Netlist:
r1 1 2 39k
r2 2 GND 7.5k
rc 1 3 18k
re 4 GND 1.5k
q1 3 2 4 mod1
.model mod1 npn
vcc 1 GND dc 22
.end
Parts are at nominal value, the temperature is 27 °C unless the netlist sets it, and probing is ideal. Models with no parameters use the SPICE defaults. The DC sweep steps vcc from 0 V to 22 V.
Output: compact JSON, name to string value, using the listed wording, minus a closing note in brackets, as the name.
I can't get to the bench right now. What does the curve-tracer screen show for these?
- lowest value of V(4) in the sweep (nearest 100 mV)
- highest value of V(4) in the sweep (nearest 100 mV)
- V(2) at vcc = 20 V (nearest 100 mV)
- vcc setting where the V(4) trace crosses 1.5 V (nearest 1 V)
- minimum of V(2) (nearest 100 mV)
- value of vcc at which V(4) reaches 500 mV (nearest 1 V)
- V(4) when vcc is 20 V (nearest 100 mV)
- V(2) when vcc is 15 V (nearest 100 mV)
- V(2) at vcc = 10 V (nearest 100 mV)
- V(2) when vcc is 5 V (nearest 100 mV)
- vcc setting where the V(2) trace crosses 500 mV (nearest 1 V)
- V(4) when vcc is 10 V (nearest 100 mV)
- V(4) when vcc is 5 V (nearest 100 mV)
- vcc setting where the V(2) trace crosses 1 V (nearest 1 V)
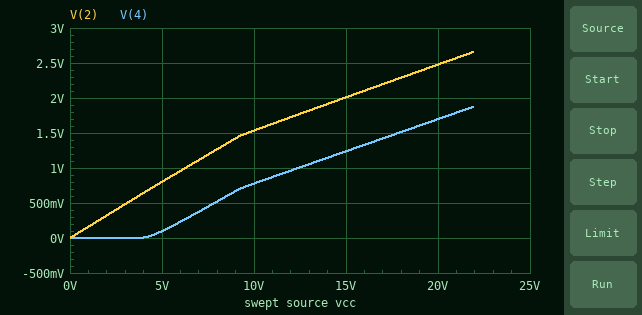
{"lowest value of V(4) in the sweep": "0 V", "highest value of V(4) in the sweep": "1.9 V", "V(2) at vcc = 20 V": "2.5 V", "vcc setting where the V(4) trace crosses 1.5 V": "18 V", "minimum of V(2)": "0 V", "value of vcc at which V(4) reaches 500 mV": "8 V", "V(4) when vcc is 20 V": "1.7 V", "V(2) when vcc is 15 V": "2.0 V", "V(2) at vcc = 10 V": "1.5 V", "V(2) when vcc is 5 V": "800 mV", "vcc setting where the V(2) trace crosses 500 mV": "3 V", "V(4) when vcc is 10 V": "800 mV", "V(4) when vcc is 5 V": "100 mV", "vcc setting where the V(2) trace crosses 1 V": "6 V"}
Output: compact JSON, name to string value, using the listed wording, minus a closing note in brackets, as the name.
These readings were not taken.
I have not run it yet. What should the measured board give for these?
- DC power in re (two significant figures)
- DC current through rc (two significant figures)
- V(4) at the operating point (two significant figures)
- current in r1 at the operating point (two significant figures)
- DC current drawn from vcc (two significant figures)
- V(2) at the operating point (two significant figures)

{"DC power in re": "2.4 mW", "DC current through rc": "1.1 mA", "V(4) at the operating point": "1.9 V", "current in r1 at the operating point": "500 µA", "DC current drawn from vcc": "1.6 mA", "V(2) at the operating point": "2.7 V"}
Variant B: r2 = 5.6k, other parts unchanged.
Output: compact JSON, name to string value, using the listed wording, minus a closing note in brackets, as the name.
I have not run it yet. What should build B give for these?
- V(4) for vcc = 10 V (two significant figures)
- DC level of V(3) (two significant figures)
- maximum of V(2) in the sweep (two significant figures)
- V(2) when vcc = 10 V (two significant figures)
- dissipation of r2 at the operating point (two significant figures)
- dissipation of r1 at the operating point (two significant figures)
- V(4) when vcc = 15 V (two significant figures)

{"V(4) for vcc = 10 V": "490 mV", "DC level of V(3)": "1.8 V", "maximum of V(2) in the sweep": "2.5 V", "V(2) when vcc = 10 V": "1.2 V", "dissipation of r2 at the operating point": "1.1 mW", "dissipation of r1 at the operating point": "9.7 mW", "V(4) when vcc = 15 V": "1.1 V"}
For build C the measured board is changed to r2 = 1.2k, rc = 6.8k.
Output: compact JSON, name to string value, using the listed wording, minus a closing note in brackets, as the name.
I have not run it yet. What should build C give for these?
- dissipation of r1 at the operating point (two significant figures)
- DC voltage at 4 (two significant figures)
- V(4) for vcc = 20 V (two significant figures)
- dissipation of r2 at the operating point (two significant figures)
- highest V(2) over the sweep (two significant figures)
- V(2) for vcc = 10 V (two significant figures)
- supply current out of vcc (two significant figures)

{"dissipation of r1 at the operating point": "12 mW", "DC voltage at 4": "11 mV", "V(4) for vcc = 20 V": "1.5 mV", "dissipation of r2 at the operating point": "360 µW", "highest V(2) over the sweep": "660 mV", "V(2) for vcc = 10 V": "300 mV", "supply current out of vcc": "550 µA"}
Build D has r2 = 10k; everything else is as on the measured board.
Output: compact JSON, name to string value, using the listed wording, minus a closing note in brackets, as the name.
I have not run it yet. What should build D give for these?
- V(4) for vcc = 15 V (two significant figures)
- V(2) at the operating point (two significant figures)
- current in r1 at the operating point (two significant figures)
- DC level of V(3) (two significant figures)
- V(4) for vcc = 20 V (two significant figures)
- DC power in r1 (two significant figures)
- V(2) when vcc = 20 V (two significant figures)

{"V(4) for vcc = 15 V": "1.3 V", "V(2) at the operating point": "2.8 V", "current in r1 at the operating point": "490 µA", "DC level of V(3)": "2.0 V", "V(4) for vcc = 20 V": "1.8 V", "DC power in r1": "9.5 mW", "V(2) when vcc = 20 V": "2.6 V"}
